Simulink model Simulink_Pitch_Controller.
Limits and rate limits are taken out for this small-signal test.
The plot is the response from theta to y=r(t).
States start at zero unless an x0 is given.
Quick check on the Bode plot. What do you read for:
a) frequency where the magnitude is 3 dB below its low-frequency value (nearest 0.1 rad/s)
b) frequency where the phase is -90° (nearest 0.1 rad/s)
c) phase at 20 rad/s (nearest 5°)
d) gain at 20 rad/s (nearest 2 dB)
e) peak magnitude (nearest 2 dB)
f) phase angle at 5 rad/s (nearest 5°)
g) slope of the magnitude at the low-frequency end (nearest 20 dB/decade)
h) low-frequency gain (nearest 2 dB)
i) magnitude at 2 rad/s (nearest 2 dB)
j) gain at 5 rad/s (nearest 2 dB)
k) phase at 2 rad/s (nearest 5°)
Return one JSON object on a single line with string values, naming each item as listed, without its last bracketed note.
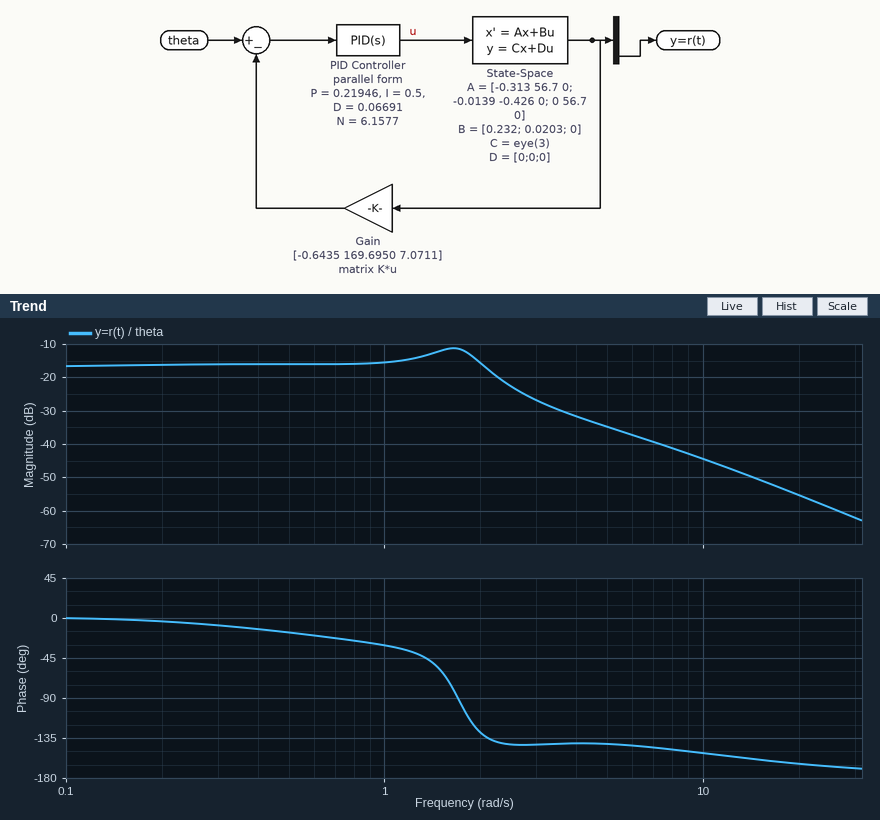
{"frequency where the magnitude is 3 dB below its low-frequency value": "2.2 rad/s", "frequency where the phase is -90°": "1.7 rad/s", "phase at 20 rad/s": "-165°", "gain at 20 rad/s": "-56 dB", "peak magnitude": "-12 dB", "phase angle at 5 rad/s": "-140°", "slope of the magnitude at the low-frequency end": "0 dB/decade", "low-frequency gain": "-16 dB", "magnitude at 2 rad/s": "-16 dB", "gain at 5 rad/s": "-34 dB", "phase at 2 rad/s": "-130°"}
